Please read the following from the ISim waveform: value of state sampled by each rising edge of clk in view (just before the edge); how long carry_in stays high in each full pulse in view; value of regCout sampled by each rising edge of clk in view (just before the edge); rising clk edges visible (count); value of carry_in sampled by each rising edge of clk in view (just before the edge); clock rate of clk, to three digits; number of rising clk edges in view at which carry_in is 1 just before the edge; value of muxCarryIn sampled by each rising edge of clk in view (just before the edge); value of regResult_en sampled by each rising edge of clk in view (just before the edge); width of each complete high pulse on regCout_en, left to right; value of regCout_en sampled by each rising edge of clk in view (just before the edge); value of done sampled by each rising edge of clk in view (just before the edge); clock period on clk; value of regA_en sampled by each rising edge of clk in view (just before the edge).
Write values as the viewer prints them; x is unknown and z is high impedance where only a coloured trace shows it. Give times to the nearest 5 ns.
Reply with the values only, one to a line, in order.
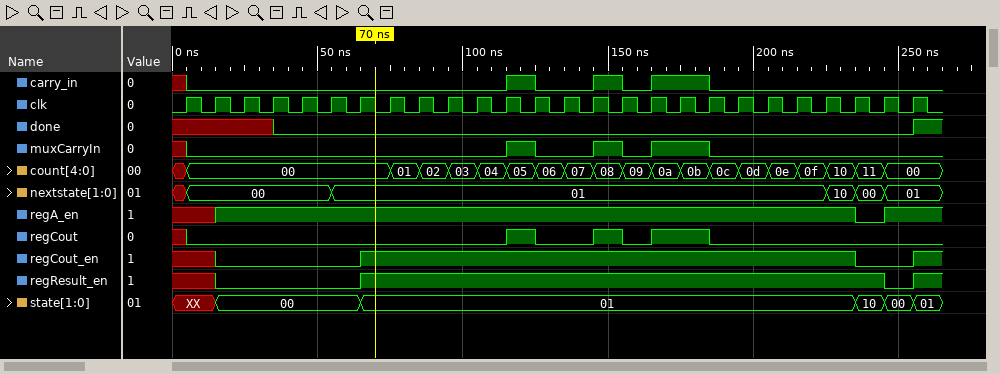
XX, XX, 00, 00, 00, 00, 00, 01, 01, 01, 01, 01, 01, 01, 01, 01, 01, 01, 01, 01, 01, 01, 01, 01, 10, 00
10 ns, 10 ns, 20 ns
x 0 0 0 0 0 0 0 0 0 0 0 1 0 0 1 0 1 1 0 0 0 0 0 0 0
26
x 0 0 0 0 0 0 0 0 0 0 0 1 0 0 1 0 1 1 0 0 0 0 0 0 0
100 MHz
4
x 0 0 0 0 0 0 0 0 0 0 0 1 0 0 1 0 1 1 0 0 0 0 0 0 0
x x 0 0 0 0 0 1 1 1 1 1 1 1 1 1 1 1 1 1 1 1 1 1 1 0
170 ns
x x 0 0 0 0 0 1 1 1 1 1 1 1 1 1 1 1 1 1 1 1 1 1 0 0
x x x x 0 0 0 0 0 0 0 0 0 0 0 0 0 0 0 0 0 0 0 0 0 0
10 ns
x x 1 1 1 1 1 1 1 1 1 1 1 1 1 1 1 1 1 1 1 1 1 1 0 1
